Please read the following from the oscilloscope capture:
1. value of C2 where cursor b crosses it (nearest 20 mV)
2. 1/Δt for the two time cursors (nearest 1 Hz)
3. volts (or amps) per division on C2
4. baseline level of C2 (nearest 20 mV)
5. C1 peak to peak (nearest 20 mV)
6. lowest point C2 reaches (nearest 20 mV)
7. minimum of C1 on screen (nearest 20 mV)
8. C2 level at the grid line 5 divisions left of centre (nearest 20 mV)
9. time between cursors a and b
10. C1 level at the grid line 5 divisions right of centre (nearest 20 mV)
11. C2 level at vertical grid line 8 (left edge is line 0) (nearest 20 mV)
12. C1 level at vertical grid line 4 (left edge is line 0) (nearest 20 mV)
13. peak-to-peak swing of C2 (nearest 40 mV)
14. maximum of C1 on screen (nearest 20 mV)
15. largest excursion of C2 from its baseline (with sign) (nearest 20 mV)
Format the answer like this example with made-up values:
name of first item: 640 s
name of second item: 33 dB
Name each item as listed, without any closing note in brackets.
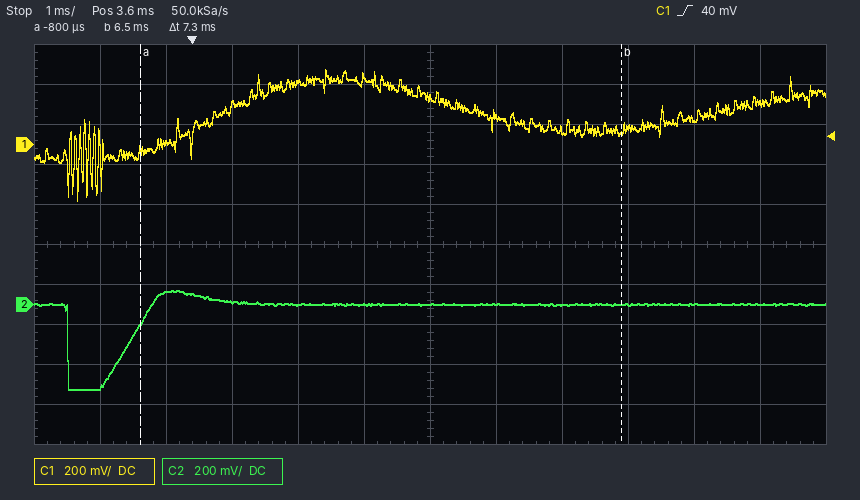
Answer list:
value of C2 where cursor b crosses it: 0 mV
1/Δt for the two time cursors: 137 Hz
volts (or amps) per division on C2: 200 mV
baseline level of C2: 0 mV
C1 peak to peak: 660 mV
lowest point C2 reaches: -420 mV
minimum of C1 on screen: -280 mV
C2 level at the grid line 5 divisions left of centre: -420 mV
time between cursors a and b: 7.3 ms
C1 level at the grid line 5 divisions right of centre: 200 mV
C2 level at vertical grid line 8 (left edge is line 0): 0 mV
C1 level at vertical grid line 4 (left edge is line 0): 300 mV
peak-to-peak swing of C2: 480 mV
maximum of C1 on screen: 380 mV
largest excursion of C2 from its baseline (with sign): -420 mV
